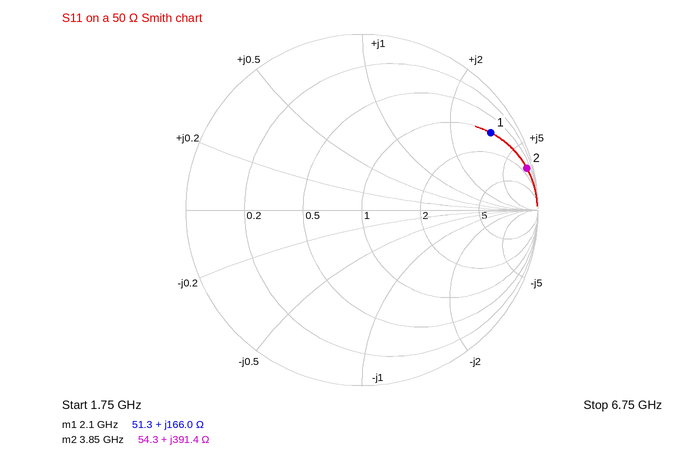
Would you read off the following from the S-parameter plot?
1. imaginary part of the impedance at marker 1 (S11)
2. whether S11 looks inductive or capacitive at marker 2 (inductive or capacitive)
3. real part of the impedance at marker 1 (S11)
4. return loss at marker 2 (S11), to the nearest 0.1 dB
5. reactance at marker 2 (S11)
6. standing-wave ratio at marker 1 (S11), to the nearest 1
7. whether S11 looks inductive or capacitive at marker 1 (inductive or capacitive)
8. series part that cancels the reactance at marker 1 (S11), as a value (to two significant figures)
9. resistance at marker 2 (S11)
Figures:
+166.0 Ω
inductive
51.3 Ω
0.3 dB
+391.4 Ω
13
inductive
460 fF
54.3 Ω
